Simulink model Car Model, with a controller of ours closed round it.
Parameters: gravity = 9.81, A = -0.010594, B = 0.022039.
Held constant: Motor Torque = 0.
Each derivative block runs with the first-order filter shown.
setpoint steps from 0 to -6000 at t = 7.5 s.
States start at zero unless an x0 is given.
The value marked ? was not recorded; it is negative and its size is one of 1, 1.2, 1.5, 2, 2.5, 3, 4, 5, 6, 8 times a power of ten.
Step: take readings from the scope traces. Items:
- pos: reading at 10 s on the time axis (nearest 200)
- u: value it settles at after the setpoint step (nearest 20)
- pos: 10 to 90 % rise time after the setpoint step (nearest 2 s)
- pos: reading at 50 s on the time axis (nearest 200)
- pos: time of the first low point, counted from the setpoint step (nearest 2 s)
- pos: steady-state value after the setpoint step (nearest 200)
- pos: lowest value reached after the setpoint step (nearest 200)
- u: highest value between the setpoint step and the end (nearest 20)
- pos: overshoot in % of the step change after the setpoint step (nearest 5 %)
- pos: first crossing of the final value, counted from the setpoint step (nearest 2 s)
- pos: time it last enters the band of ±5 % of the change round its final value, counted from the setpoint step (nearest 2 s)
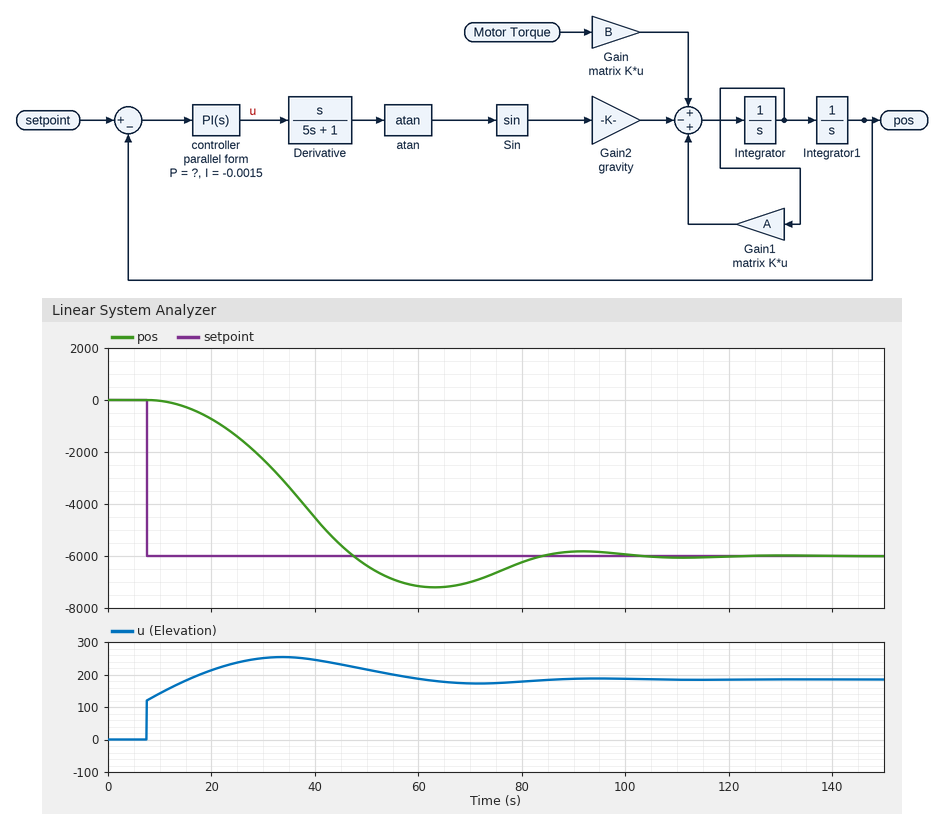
0
180
26 s
-6400
56 s
-6000
-7200
260
20 %
40 s
72 s
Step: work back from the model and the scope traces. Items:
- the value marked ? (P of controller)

-0.02
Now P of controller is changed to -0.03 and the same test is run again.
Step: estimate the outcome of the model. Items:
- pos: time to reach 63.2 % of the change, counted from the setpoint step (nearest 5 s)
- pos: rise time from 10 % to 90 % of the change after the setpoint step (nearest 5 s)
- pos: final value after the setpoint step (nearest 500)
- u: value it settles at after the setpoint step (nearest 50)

30 s
30 s
-6000
250
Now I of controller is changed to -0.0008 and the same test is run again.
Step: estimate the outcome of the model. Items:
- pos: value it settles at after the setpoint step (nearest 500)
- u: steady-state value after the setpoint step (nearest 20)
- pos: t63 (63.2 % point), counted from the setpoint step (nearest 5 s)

-6000
140
30 s
